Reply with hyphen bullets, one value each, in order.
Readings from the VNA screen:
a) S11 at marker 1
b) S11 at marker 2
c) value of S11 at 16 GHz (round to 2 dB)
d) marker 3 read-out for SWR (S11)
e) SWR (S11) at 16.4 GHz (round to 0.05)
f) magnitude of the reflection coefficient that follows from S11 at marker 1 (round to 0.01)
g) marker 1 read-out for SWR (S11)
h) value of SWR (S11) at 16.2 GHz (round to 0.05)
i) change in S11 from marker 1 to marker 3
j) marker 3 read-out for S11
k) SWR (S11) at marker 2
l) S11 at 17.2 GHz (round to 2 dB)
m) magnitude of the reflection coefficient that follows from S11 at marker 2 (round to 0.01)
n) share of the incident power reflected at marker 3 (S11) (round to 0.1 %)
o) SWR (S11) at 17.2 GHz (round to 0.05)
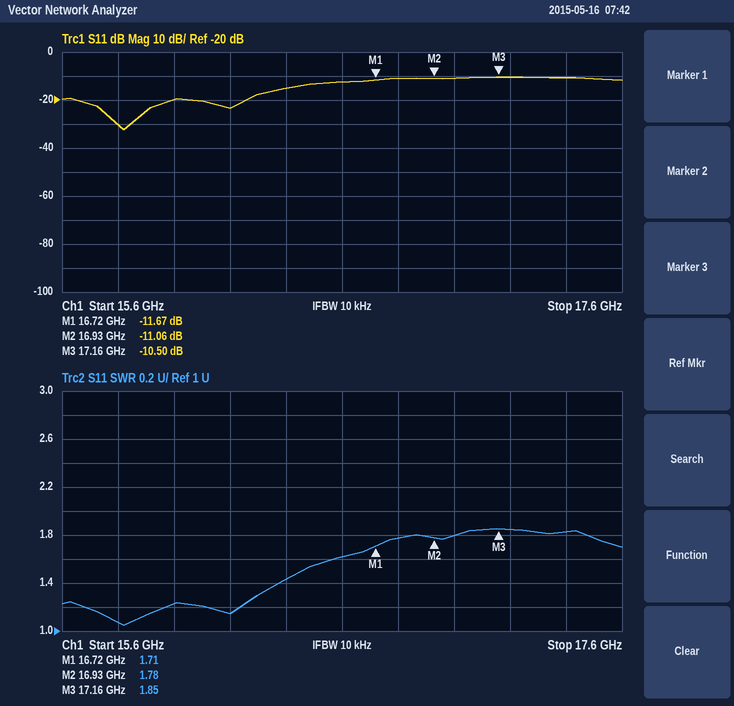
- -11.67 dB
- -11.06 dB
- -20 dB
- 1.85
- 1.45
- 0.26
- 1.71
- 1.15
- 1.17 dB
- -10.50 dB
- 1.78
- -10 dB
- 0.28
- 8.9 %
- 1.85
